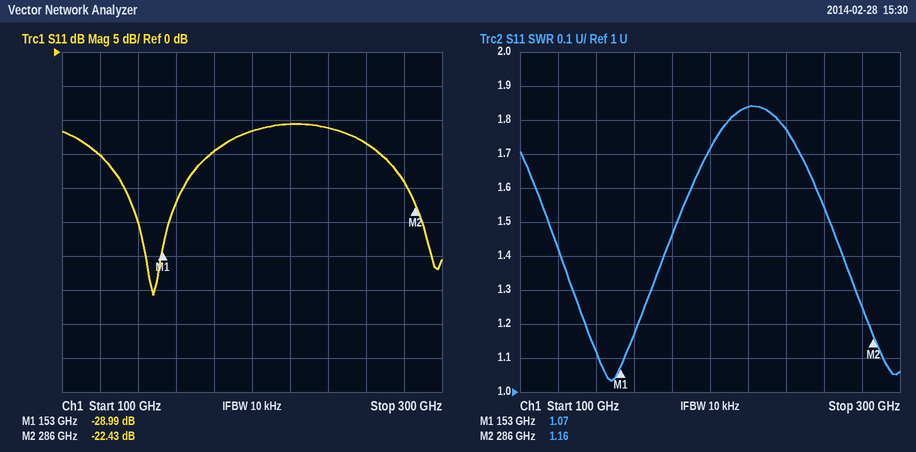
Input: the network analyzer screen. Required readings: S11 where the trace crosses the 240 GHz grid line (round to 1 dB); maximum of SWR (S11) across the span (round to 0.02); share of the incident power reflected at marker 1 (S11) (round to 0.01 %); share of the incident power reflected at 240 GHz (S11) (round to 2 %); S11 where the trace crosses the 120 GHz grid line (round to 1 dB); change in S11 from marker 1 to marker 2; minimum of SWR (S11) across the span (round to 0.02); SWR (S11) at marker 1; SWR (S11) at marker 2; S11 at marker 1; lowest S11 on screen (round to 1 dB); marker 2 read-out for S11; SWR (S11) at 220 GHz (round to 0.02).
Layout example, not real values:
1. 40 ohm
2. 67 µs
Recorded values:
1. -11 dB
2. 1.84
3. 0.13 %
4. 8 %
5. -15 dB
6. 6.56 dB
7. 1.04
8. 1.07
9. 1.16
10. -28.99 dB
11. -36 dB
12. -22.43 dB
13. 1.84
